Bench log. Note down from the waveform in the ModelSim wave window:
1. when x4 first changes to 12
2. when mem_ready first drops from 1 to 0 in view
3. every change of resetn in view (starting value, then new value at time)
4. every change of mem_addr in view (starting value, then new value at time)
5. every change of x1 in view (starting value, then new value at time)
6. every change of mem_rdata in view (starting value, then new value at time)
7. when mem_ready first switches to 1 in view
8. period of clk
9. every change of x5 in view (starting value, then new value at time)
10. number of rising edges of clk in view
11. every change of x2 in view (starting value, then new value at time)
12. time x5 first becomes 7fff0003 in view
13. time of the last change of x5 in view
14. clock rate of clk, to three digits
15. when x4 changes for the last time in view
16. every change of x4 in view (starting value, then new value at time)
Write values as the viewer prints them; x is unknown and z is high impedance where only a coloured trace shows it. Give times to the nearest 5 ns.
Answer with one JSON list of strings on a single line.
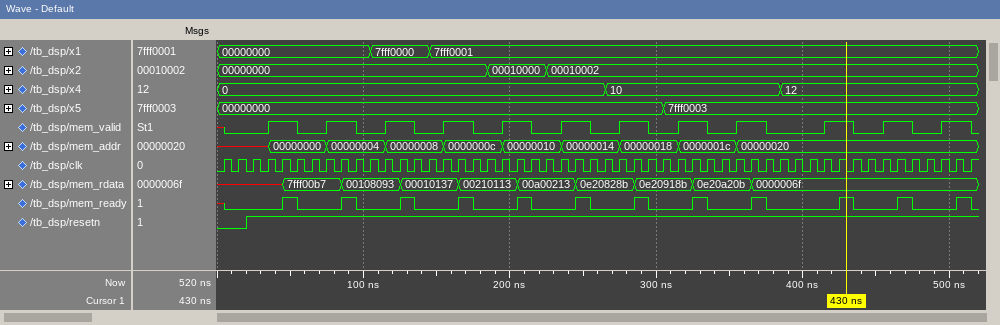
["385 ns", "55 ns", "0, 1 at 20 ns", "x, 00000000 at 35 ns, 00000004 at 75 ns, 00000008 at 115 ns, 0000000c at 155 ns, 00000010 at 195 ns, 00000014 at 235 ns, 00000018 at 275 ns, 0000001c at 315 ns, 00000020 at 355 ns", "00000000, 7fff0000 at 105 ns, 7fff0001 at 145 ns", "x, 7fff00b7 at 45 ns, 00108093 at 85 ns, 00010137 at 125 ns, 00210113 at 165 ns, 00a00213 at 205 ns, 0e20828b at 245 ns, 0e20918b at 285 ns, 0e20a20b at 325 ns, 0000006f at 365 ns", "45 ns", "10 ns", "00000000, 7fff0003 at 305 ns", "52", "00000000, 00010000 at 185 ns, 00010002 at 225 ns", "305 ns", "305 ns", "100 MHz", "385 ns", "0, 10 at 265 ns, 12 at 385 ns"]
